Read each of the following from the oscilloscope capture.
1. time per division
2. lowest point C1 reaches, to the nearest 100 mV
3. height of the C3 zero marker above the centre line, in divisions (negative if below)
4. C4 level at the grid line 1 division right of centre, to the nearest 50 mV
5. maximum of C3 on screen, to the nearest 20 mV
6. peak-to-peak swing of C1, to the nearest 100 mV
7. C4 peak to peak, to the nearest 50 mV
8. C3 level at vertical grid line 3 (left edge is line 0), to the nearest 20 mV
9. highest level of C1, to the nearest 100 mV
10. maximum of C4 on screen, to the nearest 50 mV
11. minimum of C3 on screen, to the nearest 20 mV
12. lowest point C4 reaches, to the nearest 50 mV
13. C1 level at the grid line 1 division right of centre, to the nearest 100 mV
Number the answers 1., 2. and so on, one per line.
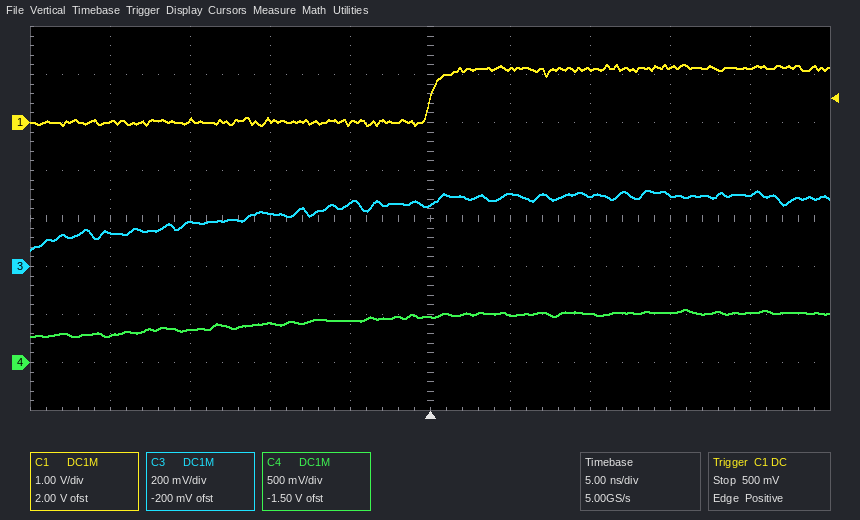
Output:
1. 5 ns
2. -100 mV
3. -1.0 div
4. 500 mV
5. 320 mV
6. 1.3 V
7. 300 mV
8. 220 mV
9. 1.2 V
10. 550 mV
11. 60 mV
12. 250 mV
13. 1.1 V
